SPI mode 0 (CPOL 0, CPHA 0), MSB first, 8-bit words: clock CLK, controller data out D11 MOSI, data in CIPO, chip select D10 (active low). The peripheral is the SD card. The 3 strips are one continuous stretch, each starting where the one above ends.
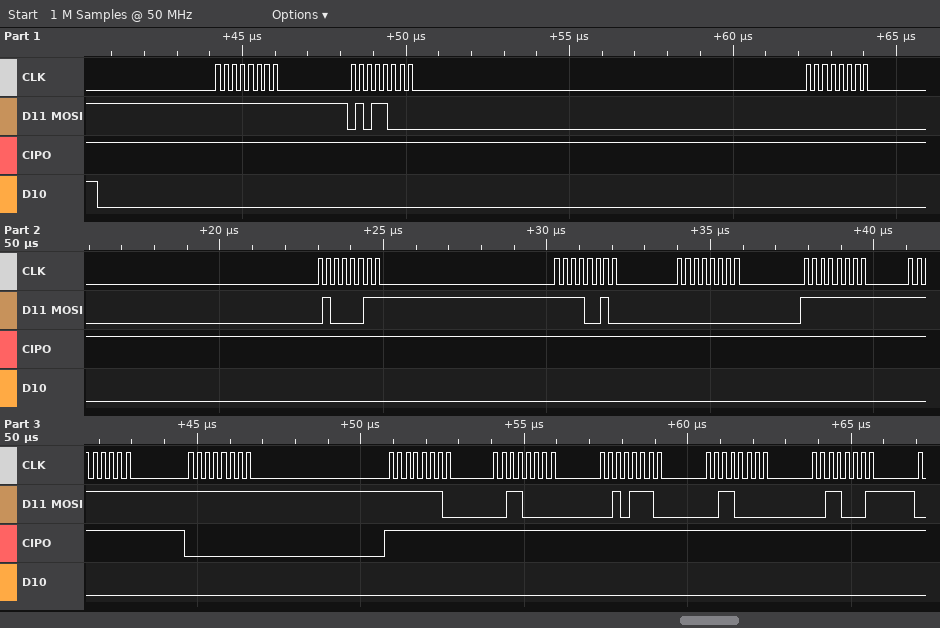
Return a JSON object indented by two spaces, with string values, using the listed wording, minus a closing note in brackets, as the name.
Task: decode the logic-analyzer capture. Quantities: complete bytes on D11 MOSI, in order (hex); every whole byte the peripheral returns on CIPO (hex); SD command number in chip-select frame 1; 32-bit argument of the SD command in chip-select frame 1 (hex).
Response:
{
  "complete bytes on D11 MOSI, in order": "0xFF 0x58 0x00 0x43 0xF2 0x00 0xFF 0xFF 0xFF 0xFE 0x30 0x2E 0x30 0x31",
  "every whole byte the peripheral returns on CIPO": "0xFF 0xFF 0xFF 0xFF 0xFF 0xFF 0xFF 0xFF 0x00 0xFF 0xFF 0xFF 0xFF 0xFF",
  "SD command number in chip-select frame 1": "CMD24",
  "32-bit argument of the SD command in chip-select frame 1": "0x0043F200"
}
